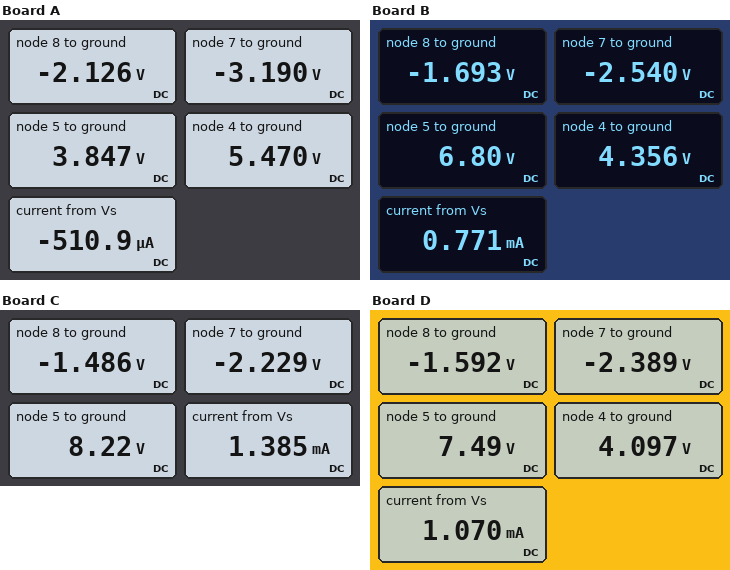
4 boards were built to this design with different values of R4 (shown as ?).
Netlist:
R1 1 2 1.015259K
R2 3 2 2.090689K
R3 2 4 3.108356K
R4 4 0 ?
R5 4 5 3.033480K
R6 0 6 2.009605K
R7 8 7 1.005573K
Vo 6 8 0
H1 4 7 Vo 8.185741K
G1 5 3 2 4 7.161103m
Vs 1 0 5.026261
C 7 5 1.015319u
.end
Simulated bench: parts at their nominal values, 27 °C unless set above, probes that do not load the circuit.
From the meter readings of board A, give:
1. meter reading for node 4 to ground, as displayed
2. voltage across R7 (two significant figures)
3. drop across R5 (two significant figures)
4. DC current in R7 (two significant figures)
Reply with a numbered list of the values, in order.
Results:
1. 5.470 V
2. 1.1 V
3. 1.6 V
4. 1.1 mA
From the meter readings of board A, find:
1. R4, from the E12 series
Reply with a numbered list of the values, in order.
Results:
1. 10 kΩ
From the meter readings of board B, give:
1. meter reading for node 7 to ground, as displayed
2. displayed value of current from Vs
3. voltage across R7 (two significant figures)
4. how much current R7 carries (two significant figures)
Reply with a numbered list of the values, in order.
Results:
1. -2.540 V
2. 0.771 mA
3. 850 mV
4. 840 µA
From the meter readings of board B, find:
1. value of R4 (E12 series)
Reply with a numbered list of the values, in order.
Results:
1. 2.7 kΩ
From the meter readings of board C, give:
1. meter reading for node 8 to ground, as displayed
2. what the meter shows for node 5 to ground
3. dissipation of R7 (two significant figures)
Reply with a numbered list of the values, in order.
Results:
1. -1.486 V
2. 8.22 V
3. 550 µW
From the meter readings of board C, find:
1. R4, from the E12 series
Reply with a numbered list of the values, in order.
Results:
1. 1.8 kΩ
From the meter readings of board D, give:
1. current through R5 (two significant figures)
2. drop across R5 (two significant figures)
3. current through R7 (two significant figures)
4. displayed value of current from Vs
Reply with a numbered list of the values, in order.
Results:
1. 1.1 mA
2. 3.4 V
3. 790 µA
4. 1.070 mA
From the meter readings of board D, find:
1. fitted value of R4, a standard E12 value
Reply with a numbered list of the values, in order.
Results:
1. 2.2 kΩ
